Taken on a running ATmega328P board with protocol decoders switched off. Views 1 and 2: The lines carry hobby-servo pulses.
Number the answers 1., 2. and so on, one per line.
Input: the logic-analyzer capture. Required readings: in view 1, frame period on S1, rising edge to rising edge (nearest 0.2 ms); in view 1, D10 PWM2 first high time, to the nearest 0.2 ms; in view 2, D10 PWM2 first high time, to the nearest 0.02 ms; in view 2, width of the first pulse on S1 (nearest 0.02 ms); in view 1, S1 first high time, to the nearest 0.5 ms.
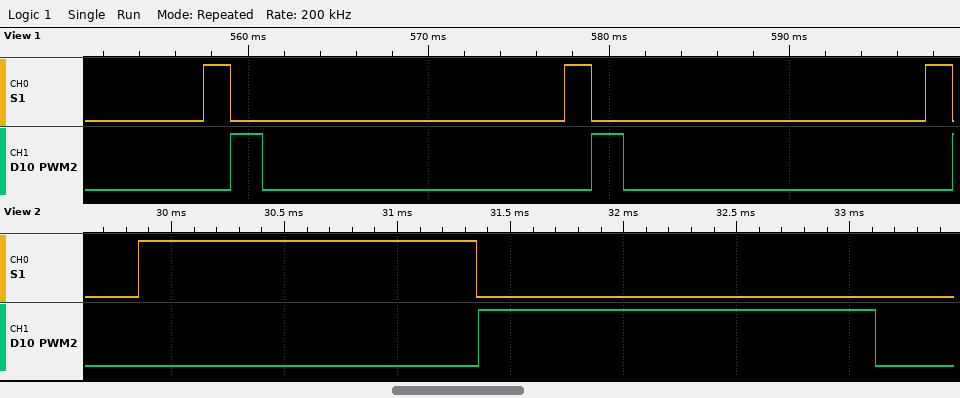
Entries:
1. 20.0 ms
2. 1.8 ms
3. 1.76 ms
4. 1.50 ms
5. 1.5 ms
